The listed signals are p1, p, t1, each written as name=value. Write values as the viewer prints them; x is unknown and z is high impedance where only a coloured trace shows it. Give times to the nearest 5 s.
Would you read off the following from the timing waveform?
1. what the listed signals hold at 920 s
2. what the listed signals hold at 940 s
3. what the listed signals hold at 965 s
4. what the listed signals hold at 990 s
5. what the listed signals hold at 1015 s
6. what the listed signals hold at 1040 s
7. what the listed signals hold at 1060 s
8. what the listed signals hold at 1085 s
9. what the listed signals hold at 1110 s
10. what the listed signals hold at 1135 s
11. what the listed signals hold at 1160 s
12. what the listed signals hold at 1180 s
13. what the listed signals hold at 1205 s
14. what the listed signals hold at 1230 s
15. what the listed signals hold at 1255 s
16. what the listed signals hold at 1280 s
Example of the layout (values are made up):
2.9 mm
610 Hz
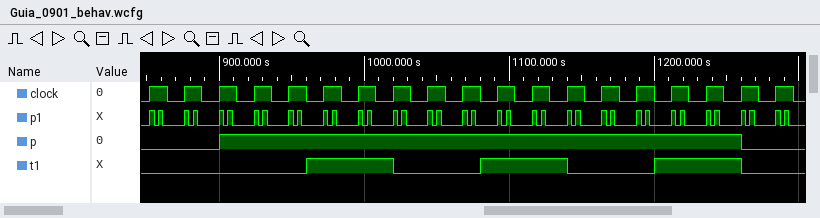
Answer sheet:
p1=0, p=1, t1=0
p1=0, p=1, t1=0
p1=0, p=1, t1=1
p1=0, p=1, t1=1
p1=0, p=1, t1=1
p1=0, p=1, t1=0
p1=0, p=1, t1=0
p1=0, p=1, t1=1
p1=0, p=1, t1=1
p1=0, p=1, t1=1
p1=0, p=1, t1=0
p1=0, p=1, t1=0
p1=0, p=1, t1=1
p1=0, p=1, t1=1
p1=0, p=1, t1=1
p1=0, p=0, t1=0
